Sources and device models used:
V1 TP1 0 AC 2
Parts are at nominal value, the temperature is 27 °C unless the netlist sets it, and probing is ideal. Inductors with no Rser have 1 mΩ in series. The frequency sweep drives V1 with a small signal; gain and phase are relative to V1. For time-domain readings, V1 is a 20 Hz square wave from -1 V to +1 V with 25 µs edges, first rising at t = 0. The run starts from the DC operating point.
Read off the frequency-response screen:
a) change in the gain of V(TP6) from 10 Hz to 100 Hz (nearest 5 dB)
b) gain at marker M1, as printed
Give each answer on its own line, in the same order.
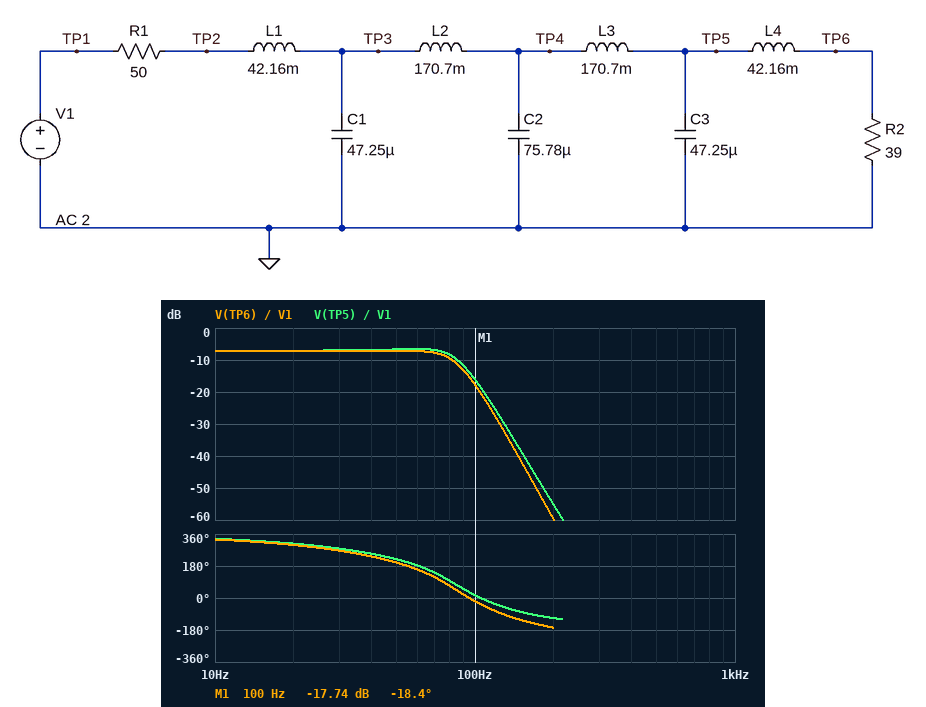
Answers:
-10 dB
-17.74 dB
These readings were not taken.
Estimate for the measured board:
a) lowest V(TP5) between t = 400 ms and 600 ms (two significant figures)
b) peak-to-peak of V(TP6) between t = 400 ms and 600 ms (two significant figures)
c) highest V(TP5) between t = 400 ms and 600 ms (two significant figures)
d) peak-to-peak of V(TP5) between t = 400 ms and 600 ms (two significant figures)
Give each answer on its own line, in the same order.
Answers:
-590 mV
1.1 V
590 mV
1.2 V
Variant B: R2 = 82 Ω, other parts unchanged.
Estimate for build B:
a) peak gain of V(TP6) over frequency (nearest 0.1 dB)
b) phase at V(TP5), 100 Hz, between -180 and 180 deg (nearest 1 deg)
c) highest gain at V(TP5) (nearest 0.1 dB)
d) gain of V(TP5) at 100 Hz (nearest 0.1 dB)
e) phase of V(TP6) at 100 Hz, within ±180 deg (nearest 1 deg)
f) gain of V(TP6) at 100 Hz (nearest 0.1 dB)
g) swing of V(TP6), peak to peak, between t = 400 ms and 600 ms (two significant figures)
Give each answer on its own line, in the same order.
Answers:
-3.9 dB
-18 deg
-3.7 dB
-15.6 dB
-36 deg
-16.1 dB
1.6 V
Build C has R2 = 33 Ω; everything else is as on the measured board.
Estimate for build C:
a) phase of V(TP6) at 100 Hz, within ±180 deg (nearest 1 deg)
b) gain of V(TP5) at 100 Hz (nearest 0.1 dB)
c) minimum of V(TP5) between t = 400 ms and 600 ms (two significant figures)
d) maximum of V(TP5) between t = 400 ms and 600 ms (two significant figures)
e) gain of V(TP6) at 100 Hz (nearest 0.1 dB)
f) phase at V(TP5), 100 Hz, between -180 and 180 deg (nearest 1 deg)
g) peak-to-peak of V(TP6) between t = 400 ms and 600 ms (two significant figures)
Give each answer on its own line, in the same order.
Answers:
-14 deg
-16.2 dB
-540 mV
540 mV
-18.4 dB
25 deg
1.0 V
